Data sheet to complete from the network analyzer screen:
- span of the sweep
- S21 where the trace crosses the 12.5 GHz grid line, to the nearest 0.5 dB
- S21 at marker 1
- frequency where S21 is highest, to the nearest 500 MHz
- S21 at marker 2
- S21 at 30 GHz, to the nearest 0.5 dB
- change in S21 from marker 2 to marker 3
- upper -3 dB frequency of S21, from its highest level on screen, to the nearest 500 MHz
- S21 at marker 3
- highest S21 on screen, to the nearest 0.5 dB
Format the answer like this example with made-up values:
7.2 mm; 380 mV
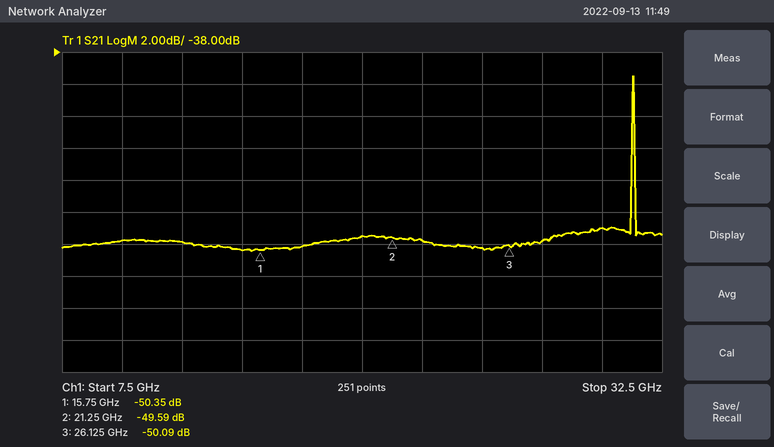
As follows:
25 GHz; -50.0 dB; -50.35 dB; 31.5 GHz; -49.59 dB; -49.0 dB; -0.50 dB; 31.5 GHz; -50.09 dB; -39.5 dB
